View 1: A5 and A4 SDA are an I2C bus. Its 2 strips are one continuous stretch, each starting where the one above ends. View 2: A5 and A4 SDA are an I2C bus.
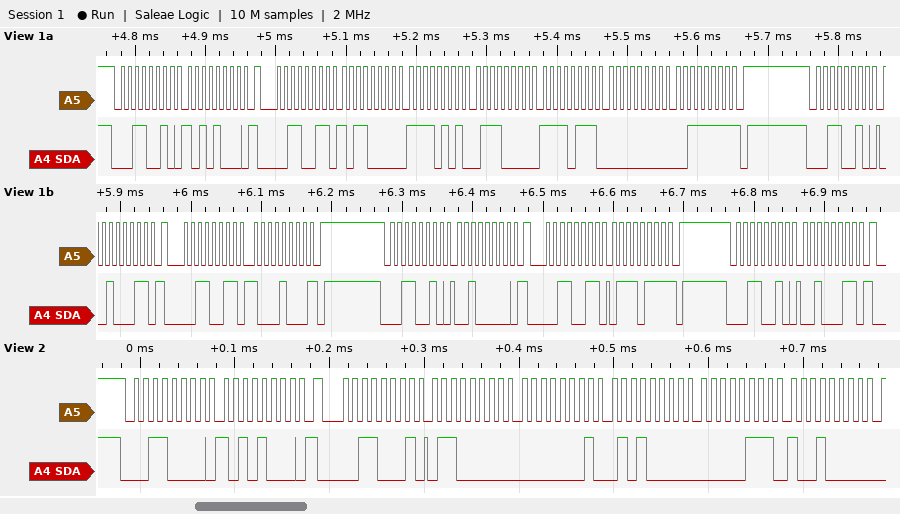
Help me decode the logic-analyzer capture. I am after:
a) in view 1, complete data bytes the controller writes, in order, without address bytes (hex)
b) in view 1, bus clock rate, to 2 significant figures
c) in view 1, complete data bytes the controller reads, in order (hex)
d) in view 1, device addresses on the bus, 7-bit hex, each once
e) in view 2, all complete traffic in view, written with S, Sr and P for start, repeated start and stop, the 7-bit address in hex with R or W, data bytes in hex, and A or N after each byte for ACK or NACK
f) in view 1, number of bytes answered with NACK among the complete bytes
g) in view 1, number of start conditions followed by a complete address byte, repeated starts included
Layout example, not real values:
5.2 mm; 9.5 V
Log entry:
A8 23 20 23; 100 kHz; B0 F5 70 F7 00 3F 88 77; 0x19; S 18W A A8 A Sr 18R A 60 A 01 A 50 A 07 A 90 A; 3; 7
